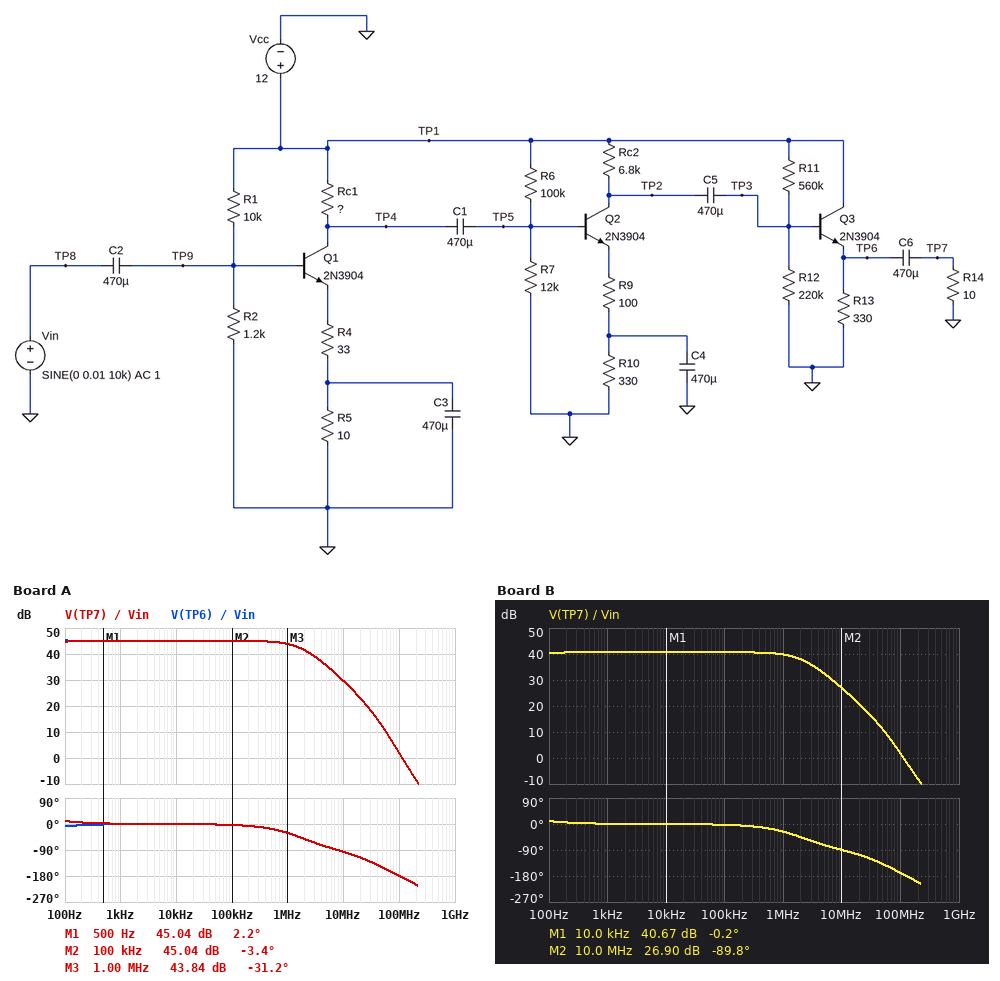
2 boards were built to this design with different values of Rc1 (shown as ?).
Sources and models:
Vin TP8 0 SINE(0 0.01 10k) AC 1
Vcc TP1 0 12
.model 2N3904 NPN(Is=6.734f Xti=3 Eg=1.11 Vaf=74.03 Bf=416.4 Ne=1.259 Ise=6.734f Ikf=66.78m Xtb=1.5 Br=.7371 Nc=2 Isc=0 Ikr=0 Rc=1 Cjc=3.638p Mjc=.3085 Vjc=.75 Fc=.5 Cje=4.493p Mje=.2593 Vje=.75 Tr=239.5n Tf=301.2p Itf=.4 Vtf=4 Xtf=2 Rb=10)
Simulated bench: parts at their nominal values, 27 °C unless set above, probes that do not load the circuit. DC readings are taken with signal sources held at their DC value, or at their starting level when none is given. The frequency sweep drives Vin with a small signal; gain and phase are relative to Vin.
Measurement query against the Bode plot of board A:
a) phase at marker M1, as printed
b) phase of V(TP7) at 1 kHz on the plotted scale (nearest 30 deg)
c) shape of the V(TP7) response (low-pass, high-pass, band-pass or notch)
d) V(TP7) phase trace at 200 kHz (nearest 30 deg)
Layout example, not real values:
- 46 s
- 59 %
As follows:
- 2.2 deg
- 0 deg
- low-pass
- 0 deg
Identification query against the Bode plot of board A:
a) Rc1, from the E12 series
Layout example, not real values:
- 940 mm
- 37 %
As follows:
- 820 Ω
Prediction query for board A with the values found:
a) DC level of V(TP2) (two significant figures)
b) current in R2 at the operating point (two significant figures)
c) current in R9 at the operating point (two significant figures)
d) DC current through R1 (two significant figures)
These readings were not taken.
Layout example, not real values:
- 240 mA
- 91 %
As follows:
- 3.8 V
- 1.0 mA
- 1.2 mA
- 1.1 mA
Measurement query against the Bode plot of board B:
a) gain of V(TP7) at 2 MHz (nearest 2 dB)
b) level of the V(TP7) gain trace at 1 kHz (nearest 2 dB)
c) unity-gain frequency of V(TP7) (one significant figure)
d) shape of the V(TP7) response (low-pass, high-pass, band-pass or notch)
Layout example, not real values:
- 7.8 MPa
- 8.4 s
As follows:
- 38 dB
- 40 dB
- 100 MHz
- low-pass
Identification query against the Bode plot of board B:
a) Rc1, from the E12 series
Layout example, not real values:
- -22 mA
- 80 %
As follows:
- 470 Ω
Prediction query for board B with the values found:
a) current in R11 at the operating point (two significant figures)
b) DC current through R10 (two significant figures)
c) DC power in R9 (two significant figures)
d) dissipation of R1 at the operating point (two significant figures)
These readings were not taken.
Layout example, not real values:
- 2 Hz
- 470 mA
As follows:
- 19 µA
- 1.2 mA
- 150 µW
- 12 mW
